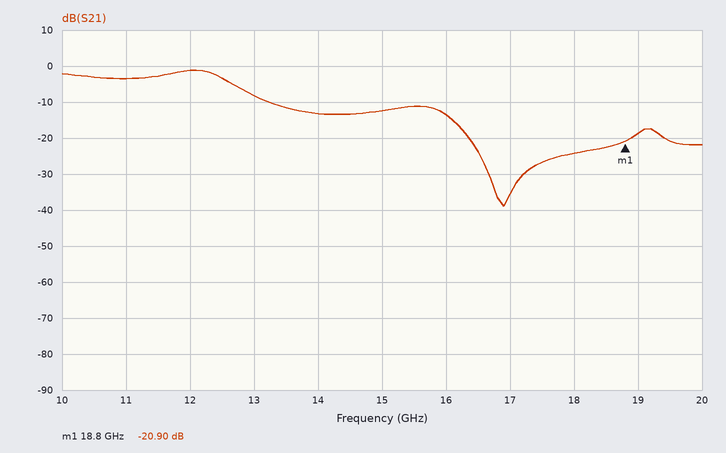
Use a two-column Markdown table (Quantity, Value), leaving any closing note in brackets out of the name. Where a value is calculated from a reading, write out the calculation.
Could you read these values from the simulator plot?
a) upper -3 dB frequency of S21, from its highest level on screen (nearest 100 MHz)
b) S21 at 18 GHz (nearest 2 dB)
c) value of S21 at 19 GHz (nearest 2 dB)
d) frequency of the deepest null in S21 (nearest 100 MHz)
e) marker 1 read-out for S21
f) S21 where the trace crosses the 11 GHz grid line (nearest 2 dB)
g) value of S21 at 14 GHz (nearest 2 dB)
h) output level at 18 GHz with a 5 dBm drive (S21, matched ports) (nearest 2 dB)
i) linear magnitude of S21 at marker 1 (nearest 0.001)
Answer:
| Quantity | Value |
|---|---|
| upper -3 dB frequency of S21, from its highest level on screen | 12.6 GHz |
| S21 at 18 GHz | -24 dB |
| value of S21 at 19 GHz | -18 dB |
| frequency of the deepest null in S21 | 16.9 GHz |
| marker 1 read-out for S21 | -20.90 dB |
| S21 where the trace crosses the 11 GHz grid line | -4 dB |
| value of S21 at 14 GHz | -14 dB |
| output level at 18 GHz with a 5 dBm drive (S21, matched ports) | 5 dBm + (-24 dB) = -20 dBm |
| linear magnitude of S21 at marker 1 | 10^(-20.9/20) ≈ 0.090 |
